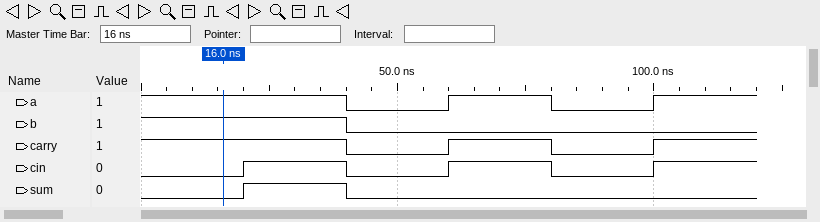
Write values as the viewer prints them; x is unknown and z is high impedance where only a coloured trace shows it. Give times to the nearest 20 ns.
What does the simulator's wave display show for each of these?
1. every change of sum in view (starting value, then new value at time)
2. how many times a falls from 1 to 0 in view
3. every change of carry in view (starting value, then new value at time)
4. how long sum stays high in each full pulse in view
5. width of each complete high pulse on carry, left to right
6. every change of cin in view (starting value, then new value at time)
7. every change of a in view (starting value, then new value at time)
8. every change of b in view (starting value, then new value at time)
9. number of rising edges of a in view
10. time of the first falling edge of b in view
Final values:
0, 1 at 20 ns, 0 at 40 ns
2
1, 0 at 40 ns, 1 at 60 ns, 0 at 80 ns, 1 at 100 ns
20 ns
20 ns
0, 1 at 20 ns, 0 at 40 ns, 1 at 60 ns, 0 at 80 ns, 1 at 100 ns
1, 0 at 40 ns, 1 at 60 ns, 0 at 80 ns, 1 at 100 ns
1, 0 at 40 ns
2
40 ns
